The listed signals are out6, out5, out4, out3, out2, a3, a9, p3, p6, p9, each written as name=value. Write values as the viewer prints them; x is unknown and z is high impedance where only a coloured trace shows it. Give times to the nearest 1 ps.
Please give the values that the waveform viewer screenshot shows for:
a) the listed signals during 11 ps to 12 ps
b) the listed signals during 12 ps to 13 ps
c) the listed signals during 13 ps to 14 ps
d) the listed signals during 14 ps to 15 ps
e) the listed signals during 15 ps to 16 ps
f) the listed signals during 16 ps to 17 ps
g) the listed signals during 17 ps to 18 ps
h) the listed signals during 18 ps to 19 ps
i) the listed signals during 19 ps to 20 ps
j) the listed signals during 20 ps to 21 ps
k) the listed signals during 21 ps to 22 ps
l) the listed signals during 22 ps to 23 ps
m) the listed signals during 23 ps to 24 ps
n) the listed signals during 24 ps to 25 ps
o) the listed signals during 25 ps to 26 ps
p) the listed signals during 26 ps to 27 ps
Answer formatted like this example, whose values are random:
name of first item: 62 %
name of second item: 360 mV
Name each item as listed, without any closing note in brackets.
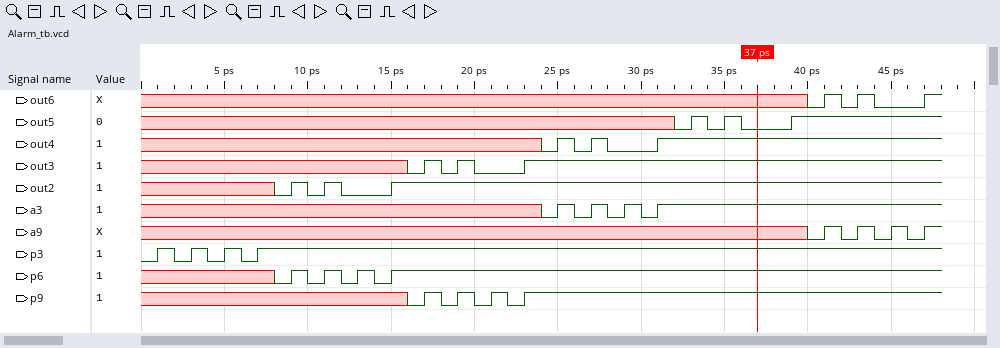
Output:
the listed signals during 11 ps to 12 ps: out6=x, out5=x, out4=x, out3=x, out2=1, a3=x, a9=x, p3=1, p6=1, p9=x
the listed signals during 12 ps to 13 ps: out6=x, out5=x, out4=x, out3=x, out2=0, a3=x, a9=x, p3=1, p6=0, p9=x
the listed signals during 13 ps to 14 ps: out6=x, out5=x, out4=x, out3=x, out2=0, a3=x, a9=x, p3=1, p6=1, p9=x
the listed signals during 14 ps to 15 ps: out6=x, out5=x, out4=x, out3=x, out2=0, a3=x, a9=x, p3=1, p6=0, p9=x
the listed signals during 15 ps to 16 ps: out6=x, out5=x, out4=x, out3=x, out2=1, a3=x, a9=x, p3=1, p6=1, p9=x
the listed signals during 16 ps to 17 ps: out6=x, out5=x, out4=x, out3=0, out2=1, a3=x, a9=x, p3=1, p6=1, p9=0
the listed signals during 17 ps to 18 ps: out6=x, out5=x, out4=x, out3=1, out2=1, a3=x, a9=x, p3=1, p6=1, p9=1
the listed signals during 18 ps to 19 ps: out6=x, out5=x, out4=x, out3=0, out2=1, a3=x, a9=x, p3=1, p6=1, p9=0
the listed signals during 19 ps to 20 ps: out6=x, out5=x, out4=x, out3=1, out2=1, a3=x, a9=x, p3=1, p6=1, p9=1
the listed signals during 20 ps to 21 ps: out6=x, out5=x, out4=x, out3=0, out2=1, a3=x, a9=x, p3=1, p6=1, p9=0
the listed signals during 21 ps to 22 ps: out6=x, out5=x, out4=x, out3=0, out2=1, a3=x, a9=x, p3=1, p6=1, p9=1
the listed signals during 22 ps to 23 ps: out6=x, out5=x, out4=x, out3=0, out2=1, a3=x, a9=x, p3=1, p6=1, p9=0
the listed signals during 23 ps to 24 ps: out6=x, out5=x, out4=x, out3=1, out2=1, a3=x, a9=x, p3=1, p6=1, p9=1
the listed signals during 24 ps to 25 ps: out6=x, out5=x, out4=0, out3=1, out2=1, a3=0, a9=x, p3=1, p6=1, p9=1
the listed signals during 25 ps to 26 ps: out6=x, out5=x, out4=1, out3=1, out2=1, a3=1, a9=x, p3=1, p6=1, p9=1
the listed signals during 26 ps to 27 ps: out6=x, out5=x, out4=0, out3=1, out2=1, a3=0, a9=x, p3=1, p6=1, p9=1
